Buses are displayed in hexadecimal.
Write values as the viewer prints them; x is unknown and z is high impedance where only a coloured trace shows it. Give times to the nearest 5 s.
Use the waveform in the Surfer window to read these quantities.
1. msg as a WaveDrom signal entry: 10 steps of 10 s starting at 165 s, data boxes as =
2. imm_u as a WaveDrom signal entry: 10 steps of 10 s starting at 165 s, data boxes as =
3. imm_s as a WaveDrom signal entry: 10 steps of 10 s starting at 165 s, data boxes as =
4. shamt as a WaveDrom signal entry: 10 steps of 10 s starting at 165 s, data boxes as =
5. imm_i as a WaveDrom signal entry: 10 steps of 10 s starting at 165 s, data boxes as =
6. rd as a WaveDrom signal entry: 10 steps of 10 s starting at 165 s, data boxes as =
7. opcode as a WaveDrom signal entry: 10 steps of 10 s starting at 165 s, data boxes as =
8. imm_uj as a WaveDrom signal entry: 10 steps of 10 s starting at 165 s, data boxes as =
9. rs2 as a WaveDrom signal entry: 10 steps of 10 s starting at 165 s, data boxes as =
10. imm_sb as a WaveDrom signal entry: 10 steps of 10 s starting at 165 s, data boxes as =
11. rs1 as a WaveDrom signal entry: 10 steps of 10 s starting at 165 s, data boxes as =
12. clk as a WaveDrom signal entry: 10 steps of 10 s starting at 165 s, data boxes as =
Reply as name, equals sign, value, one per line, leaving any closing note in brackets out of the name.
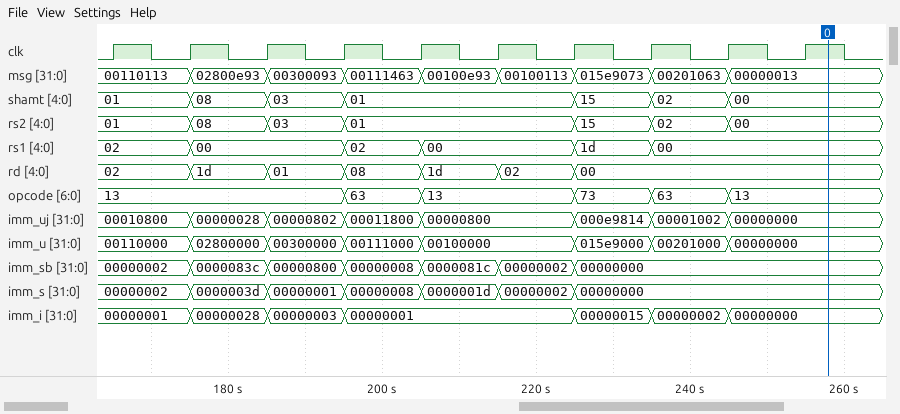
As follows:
msg as a WaveDrom signal entry: 10 steps of 10 s starting at 165 s, data boxes as = = {name: 'msg', wave: '=========.', data: '00110113 02800e93 00300093 00111463 00100e93 00100113 015e9073 00201063 00000013'}
imm_u as a WaveDrom signal entry: 10 steps of 10 s starting at 165 s, data boxes as = = {name: 'imm_u', wave: '=====.===.', data: '00110000 02800000 00300000 00111000 00100000 015e9000 00201000 00000000'}
imm_s as a WaveDrom signal entry: 10 steps of 10 s starting at 165 s, data boxes as = = {name: 'imm_s', wave: '=======...', data: '00000002 0000003d 00000001 00000008 0000001d 00000002 00000000'}
shamt as a WaveDrom signal entry: 10 steps of 10 s starting at 165 s, data boxes as = = {name: 'shamt', wave: '====..===.', data: '01 08 03 01 15 02 00'}
imm_i as a WaveDrom signal entry: 10 steps of 10 s starting at 165 s, data boxes as = = {name: 'imm_i', wave: '====..===.', data: '00000001 00000028 00000003 00000001 00000015 00000002 00000000'}
rd as a WaveDrom signal entry: 10 steps of 10 s starting at 165 s, data boxes as = = {name: 'rd', wave: '=======...', data: '02 1d 01 08 1d 02 00'}
opcode as a WaveDrom signal entry: 10 steps of 10 s starting at 165 s, data boxes as = = {name: 'opcode', wave: '=..==.===.', data: '13 63 13 73 63 13'}
imm_uj as a WaveDrom signal entry: 10 steps of 10 s starting at 165 s, data boxes as = = {name: 'imm_uj', wave: '=====.===.', data: '00010800 00000028 00000802 00011800 00000800 000e9814 00001002 00000000'}
rs2 as a WaveDrom signal entry: 10 steps of 10 s starting at 165 s, data boxes as = = {name: 'rs2', wave: '====..===.', data: '01 08 03 01 15 02 00'}
imm_sb as a WaveDrom signal entry: 10 steps of 10 s starting at 165 s, data boxes as = = {name: 'imm_sb', wave: '=======...', data: '00000002 0000083c 00000800 00000008 0000081c 00000002 00000000'}
rs1 as a WaveDrom signal entry: 10 steps of 10 s starting at 165 s, data boxes as = = {name: 'rs1', wave: '==.==.==..', data: '02 00 02 00 1d 00'}
clk as a WaveDrom signal entry: 10 steps of 10 s starting at 165 s, data boxes as = = {name: 'clk', wave: 'p.........'}
